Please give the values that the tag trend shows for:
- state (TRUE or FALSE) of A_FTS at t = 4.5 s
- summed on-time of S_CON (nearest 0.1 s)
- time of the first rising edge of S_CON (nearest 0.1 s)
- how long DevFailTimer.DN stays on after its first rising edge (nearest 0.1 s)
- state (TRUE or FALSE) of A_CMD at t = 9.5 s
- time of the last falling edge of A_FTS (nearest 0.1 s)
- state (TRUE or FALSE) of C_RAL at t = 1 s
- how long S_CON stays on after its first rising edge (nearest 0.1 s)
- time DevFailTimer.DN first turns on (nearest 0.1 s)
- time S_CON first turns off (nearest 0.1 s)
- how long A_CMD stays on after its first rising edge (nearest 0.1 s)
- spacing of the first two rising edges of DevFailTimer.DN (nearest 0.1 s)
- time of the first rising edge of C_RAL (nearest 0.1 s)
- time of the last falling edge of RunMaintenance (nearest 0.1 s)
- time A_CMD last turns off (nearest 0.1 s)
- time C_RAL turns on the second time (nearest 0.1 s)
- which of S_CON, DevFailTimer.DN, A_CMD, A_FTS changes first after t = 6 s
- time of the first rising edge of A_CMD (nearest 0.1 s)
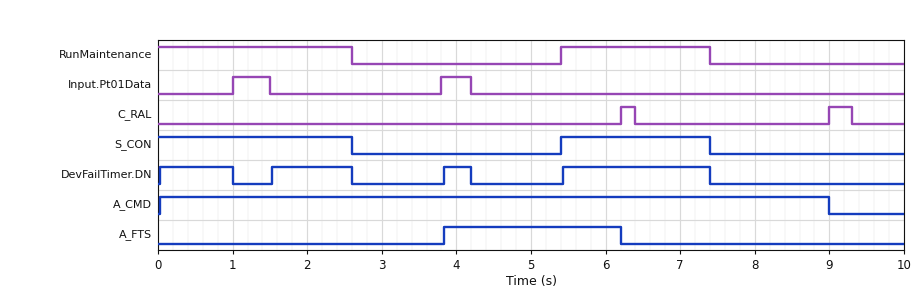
TRUE
4.6 s
5.4 s
1.0 s
FALSE
6.2 s
FALSE
2.0 s
0.0 s
2.6 s
9.0 s
1.5 s
6.2 s
7.4 s
9.0 s
9.0 s
A_FTS
0.0 s
